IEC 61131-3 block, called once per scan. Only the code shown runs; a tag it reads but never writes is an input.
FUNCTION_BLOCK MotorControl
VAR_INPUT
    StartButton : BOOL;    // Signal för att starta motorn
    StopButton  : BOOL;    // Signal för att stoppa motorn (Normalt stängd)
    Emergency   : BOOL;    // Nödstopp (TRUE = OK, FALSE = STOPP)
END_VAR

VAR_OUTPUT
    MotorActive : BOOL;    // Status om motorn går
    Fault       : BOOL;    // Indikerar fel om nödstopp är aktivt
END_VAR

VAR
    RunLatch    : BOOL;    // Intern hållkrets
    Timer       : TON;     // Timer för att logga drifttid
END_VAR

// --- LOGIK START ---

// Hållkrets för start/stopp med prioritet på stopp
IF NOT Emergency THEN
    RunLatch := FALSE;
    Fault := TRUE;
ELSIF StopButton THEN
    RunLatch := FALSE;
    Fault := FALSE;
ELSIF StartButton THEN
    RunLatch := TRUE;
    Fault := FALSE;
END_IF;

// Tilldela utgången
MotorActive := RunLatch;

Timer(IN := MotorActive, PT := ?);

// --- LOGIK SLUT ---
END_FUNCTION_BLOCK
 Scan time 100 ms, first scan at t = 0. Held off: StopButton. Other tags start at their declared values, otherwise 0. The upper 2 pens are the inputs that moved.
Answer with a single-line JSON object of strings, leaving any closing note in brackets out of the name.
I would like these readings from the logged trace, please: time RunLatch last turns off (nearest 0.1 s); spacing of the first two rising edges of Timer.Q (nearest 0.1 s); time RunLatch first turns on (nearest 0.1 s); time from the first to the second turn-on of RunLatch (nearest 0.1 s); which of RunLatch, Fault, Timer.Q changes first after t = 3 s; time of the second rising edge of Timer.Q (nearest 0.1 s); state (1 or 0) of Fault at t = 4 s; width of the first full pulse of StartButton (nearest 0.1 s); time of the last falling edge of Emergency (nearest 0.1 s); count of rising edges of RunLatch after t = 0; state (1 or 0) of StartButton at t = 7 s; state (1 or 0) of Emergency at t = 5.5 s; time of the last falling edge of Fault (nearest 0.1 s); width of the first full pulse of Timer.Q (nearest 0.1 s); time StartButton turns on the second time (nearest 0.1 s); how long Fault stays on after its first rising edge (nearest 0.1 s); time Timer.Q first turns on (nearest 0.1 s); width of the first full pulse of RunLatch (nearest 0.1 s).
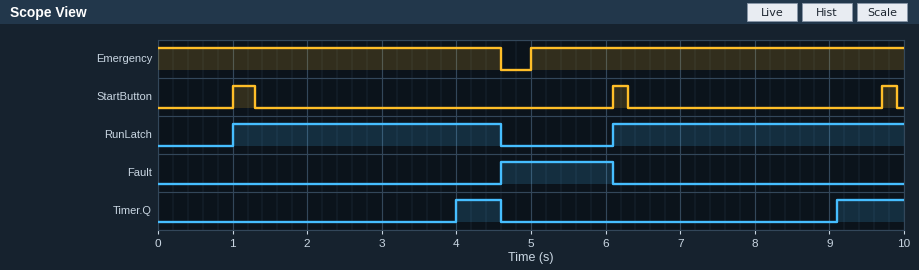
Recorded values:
{"time RunLatch last turns off": "4.6 s", "spacing of the first two rising edges of Timer.Q": "5.1 s", "time RunLatch first turns on": "1.0 s", "time from the first to the second turn-on of RunLatch": "5.1 s", "which of RunLatch, Fault, Timer.Q changes first after t = 3 s": "Timer.Q", "time of the second rising edge of Timer.Q": "9.1 s", "state (1 or 0) of Fault at t = 4 s": "0", "width of the first full pulse of StartButton": "0.3 s", "time of the last falling edge of Emergency": "4.6 s", "count of rising edges of RunLatch after t = 0": "2", "state (1 or 0) of StartButton at t = 7 s": "0", "state (1 or 0) of Emergency at t = 5.5 s": "1", "time of the last falling edge of Fault": "6.1 s", "width of the first full pulse of Timer.Q": "0.6 s", "time StartButton turns on the second time": "6.1 s", "how long Fault stays on after its first rising edge": "1.5 s", "time Timer.Q first turns on": "4.0 s", "width of the first full pulse of RunLatch": "3.6 s"}
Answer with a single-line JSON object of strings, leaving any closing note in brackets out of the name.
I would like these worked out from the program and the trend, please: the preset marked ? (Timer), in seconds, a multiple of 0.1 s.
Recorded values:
{"the preset marked ? (Timer), in seconds, a multiple of 0.1 s": "3.0 s"}
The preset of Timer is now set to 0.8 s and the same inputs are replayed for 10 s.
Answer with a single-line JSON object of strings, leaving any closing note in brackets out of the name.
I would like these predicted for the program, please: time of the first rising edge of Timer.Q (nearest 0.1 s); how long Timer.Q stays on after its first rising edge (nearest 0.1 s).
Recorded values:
{"time of the first rising edge of Timer.Q": "1.8 s", "how long Timer.Q stays on after its first rising edge": "2.8 s"}
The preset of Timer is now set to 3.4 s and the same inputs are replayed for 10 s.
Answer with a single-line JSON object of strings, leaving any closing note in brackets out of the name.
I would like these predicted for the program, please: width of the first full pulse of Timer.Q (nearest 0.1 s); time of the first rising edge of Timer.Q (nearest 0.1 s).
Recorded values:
{"width of the first full pulse of Timer.Q": "0.2 s", "time of the first rising edge of Timer.Q": "4.4 s"}
